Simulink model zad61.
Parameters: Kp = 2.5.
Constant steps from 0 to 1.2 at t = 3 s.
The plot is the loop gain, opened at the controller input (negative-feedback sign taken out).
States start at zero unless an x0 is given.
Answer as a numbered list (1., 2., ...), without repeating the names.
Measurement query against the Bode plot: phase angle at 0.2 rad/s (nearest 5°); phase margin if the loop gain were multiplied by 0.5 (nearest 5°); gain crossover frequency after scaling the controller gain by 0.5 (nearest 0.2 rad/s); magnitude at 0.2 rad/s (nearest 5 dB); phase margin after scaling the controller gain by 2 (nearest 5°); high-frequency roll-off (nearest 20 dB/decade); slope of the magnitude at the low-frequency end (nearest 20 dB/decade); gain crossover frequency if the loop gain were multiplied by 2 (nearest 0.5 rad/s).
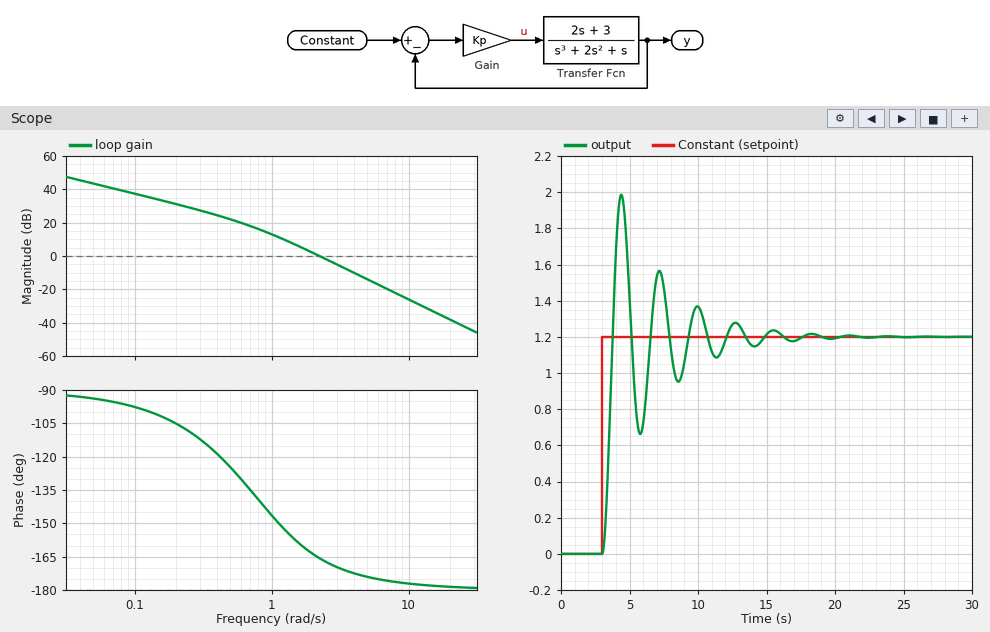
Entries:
1. -105°
2. 20°
3. 1.6 rad/s
4. 30 dB
5. 10°
6. -40 dB/decade
7. -20 dB/decade
8. 3.0 rad/s
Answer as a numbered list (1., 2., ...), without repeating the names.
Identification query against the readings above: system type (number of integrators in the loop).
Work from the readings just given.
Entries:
1. 1
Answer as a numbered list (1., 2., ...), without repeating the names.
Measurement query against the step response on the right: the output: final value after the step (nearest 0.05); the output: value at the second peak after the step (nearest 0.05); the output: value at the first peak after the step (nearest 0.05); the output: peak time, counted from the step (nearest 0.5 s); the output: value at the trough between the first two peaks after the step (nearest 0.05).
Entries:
1. 1.20
2. 1.55
3. 2.00
4. 1.5 s
5. 0.65
